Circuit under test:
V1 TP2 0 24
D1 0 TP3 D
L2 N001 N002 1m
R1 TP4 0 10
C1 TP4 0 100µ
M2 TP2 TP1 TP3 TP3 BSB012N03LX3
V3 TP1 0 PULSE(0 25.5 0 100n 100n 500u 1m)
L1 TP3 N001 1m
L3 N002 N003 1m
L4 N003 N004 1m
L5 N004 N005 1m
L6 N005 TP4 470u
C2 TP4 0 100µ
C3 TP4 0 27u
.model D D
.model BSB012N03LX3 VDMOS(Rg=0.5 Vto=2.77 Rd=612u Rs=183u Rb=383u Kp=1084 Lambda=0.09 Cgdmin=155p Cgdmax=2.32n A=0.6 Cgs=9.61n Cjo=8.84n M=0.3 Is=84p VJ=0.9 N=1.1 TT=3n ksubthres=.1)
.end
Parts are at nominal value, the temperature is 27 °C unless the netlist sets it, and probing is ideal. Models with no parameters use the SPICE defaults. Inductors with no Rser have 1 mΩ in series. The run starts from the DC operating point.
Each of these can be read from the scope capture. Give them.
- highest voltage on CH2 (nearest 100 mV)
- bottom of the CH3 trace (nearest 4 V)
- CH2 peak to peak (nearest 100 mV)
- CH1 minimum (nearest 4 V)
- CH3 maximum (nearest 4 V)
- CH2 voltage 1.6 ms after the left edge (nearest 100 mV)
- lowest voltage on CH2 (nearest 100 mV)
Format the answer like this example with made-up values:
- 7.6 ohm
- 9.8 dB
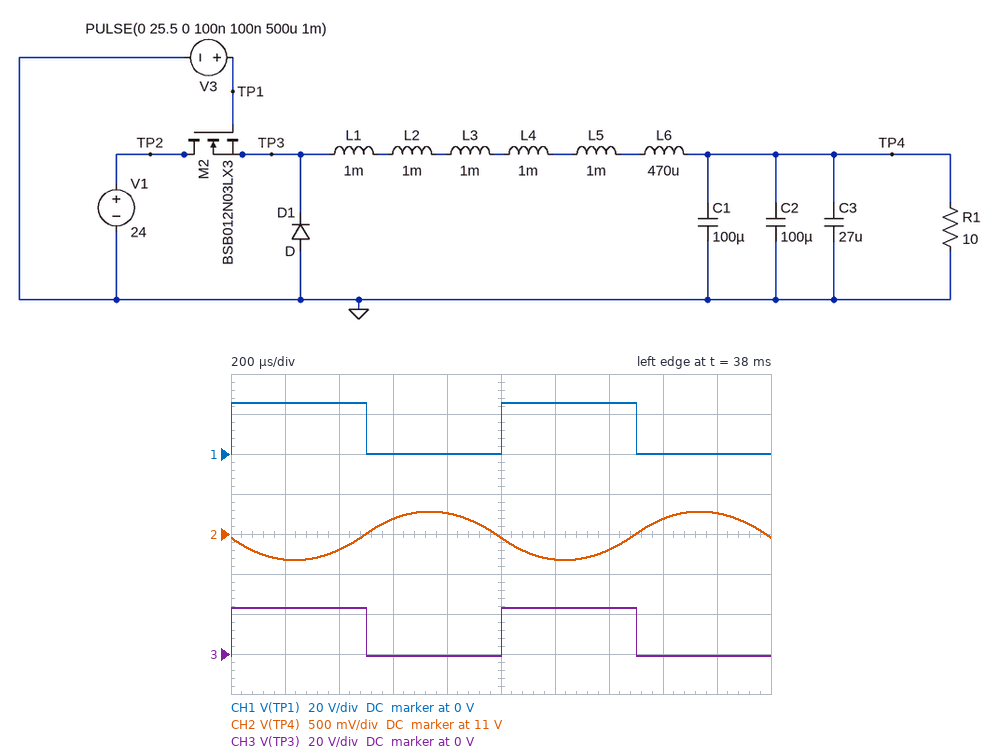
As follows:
- 11.3 V
- 0 V
- 600 mV
- 0 V
- 24 V
- 11.2 V
- 10.7 V
